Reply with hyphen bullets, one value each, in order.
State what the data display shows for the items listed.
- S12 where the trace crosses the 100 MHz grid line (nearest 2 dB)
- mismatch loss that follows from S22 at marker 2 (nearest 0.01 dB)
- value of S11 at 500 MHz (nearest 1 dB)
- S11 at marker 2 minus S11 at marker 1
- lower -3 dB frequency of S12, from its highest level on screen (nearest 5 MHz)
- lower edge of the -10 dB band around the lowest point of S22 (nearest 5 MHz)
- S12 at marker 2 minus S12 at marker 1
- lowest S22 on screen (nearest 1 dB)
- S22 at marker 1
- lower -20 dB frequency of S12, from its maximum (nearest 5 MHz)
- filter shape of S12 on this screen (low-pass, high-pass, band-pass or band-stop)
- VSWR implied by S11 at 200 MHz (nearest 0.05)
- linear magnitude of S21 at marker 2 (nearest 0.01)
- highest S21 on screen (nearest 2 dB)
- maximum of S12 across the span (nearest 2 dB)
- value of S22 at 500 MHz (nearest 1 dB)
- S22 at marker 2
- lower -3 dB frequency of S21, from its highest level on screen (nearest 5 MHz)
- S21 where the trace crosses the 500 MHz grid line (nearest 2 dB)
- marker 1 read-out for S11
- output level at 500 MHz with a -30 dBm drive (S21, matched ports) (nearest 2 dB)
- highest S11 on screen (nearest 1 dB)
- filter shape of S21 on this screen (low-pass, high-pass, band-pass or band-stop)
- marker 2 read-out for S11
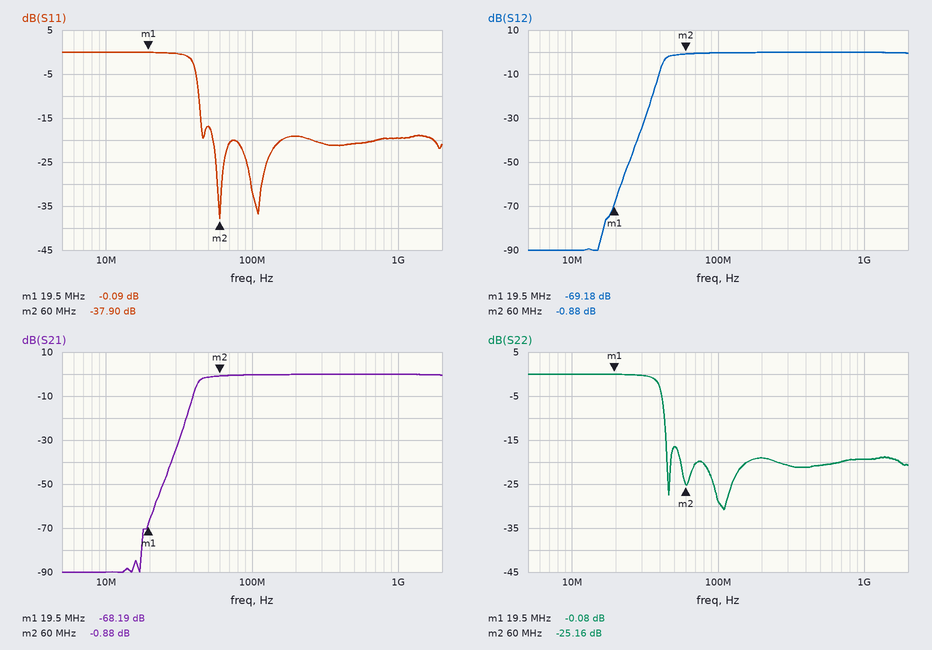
- 0 dB
- 0.01 dB
- -21 dB
- -37.81 dB
- 45 MHz
- 45 MHz
- 68.30 dB
- -31 dB
- -0.08 dB
- 35 MHz
- high-pass
- 1.25
- 0.90
- 0 dB
- 0 dB
- -21 dB
- -25.16 dB
- 45 MHz
- 0 dB
- -0.09 dB
- -30 dBm
- 0 dB
- high-pass
- -37.90 dB
